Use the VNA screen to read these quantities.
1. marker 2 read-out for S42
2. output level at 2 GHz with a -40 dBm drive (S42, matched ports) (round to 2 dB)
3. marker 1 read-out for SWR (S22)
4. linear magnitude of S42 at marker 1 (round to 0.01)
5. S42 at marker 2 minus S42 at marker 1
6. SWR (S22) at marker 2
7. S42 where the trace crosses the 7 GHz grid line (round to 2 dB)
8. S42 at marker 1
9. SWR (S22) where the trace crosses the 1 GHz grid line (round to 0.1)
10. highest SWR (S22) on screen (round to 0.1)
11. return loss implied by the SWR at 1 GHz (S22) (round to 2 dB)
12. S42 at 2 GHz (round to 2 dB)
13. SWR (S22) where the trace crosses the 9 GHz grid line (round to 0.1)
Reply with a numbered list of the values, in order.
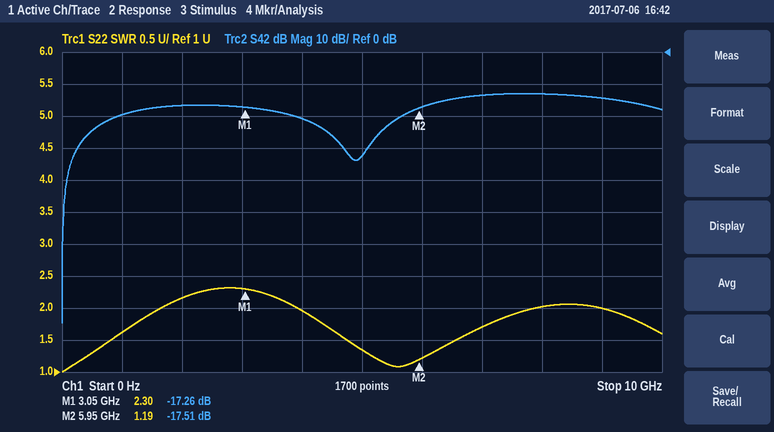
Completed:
1. -17.51 dB
2. -56 dBm
3. 2.30
4. 0.14
5. -0.25 dB
6. 1.19
7. -14 dB
8. -17.26 dB
9. 1.6
10. 2.3
11. 12 dB
12. -16 dB
13. 2.0
